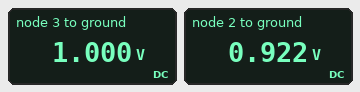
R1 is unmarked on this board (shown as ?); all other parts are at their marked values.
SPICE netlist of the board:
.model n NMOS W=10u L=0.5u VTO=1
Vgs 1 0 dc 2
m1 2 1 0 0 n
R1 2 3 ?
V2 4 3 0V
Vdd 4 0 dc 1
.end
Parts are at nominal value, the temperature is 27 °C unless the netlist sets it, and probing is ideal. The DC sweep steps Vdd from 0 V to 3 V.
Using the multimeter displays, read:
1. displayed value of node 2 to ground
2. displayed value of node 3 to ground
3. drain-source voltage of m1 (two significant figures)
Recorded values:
0.922 V
1.000 V
920 mV
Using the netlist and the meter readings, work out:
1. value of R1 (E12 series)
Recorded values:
390 Ω
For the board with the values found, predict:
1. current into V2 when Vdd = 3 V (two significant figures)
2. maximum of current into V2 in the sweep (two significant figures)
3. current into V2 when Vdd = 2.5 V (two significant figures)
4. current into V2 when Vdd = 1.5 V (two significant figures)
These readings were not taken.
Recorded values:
200 µA
200 µA
200 µA
200 µA
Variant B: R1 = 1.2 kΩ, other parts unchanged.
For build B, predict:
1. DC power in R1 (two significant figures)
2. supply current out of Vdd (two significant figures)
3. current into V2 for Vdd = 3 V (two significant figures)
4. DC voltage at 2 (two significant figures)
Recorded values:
43 µW
190 µA
200 µA
770 mV
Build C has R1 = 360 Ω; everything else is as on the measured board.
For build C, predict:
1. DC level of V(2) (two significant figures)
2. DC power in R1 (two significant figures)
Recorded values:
930 mV
14 µW
